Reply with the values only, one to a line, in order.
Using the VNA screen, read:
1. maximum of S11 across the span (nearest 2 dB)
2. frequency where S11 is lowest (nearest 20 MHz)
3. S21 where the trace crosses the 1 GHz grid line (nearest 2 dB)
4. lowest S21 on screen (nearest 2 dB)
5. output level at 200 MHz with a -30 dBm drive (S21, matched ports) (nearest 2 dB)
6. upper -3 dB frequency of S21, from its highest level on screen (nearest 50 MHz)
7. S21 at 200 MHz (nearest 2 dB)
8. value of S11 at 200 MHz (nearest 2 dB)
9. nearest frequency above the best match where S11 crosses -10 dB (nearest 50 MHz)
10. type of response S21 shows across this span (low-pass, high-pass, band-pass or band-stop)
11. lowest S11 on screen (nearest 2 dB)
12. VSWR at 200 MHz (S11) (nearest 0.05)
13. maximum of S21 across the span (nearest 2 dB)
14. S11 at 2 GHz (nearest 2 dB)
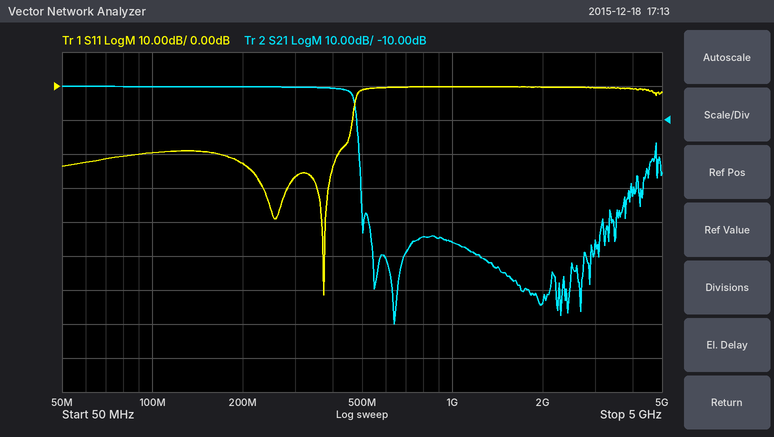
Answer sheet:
0 dB
380 MHz
-46 dB
-70 dB
-30 dBm
450 MHz
0 dB
-22 dB
450 MHz
low-pass
-62 dB
1.15
0 dB
0 dB
